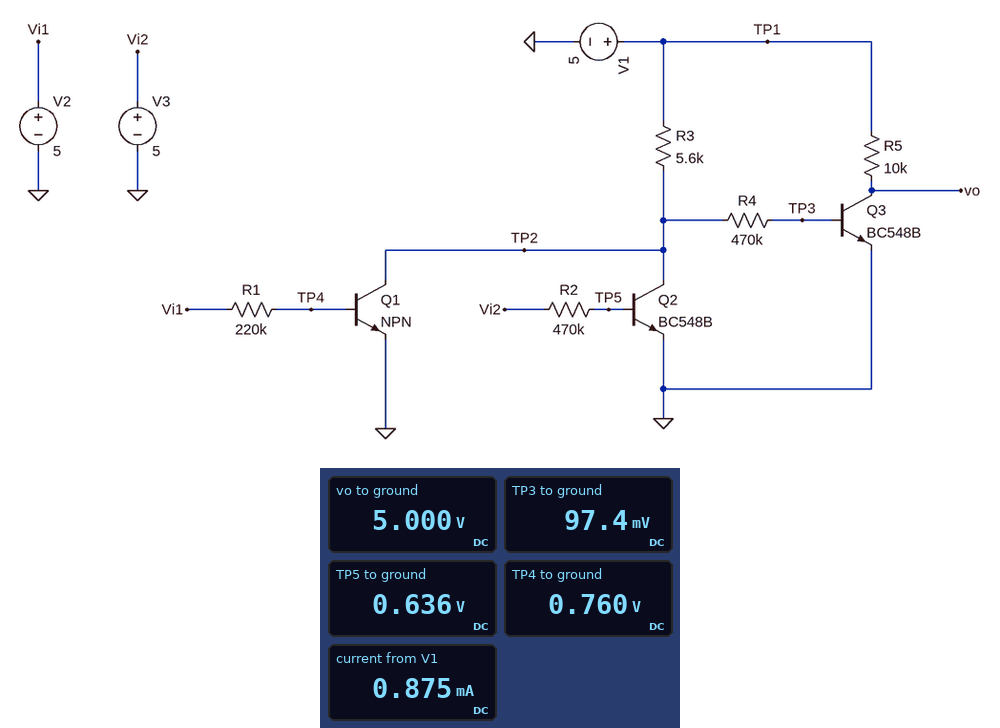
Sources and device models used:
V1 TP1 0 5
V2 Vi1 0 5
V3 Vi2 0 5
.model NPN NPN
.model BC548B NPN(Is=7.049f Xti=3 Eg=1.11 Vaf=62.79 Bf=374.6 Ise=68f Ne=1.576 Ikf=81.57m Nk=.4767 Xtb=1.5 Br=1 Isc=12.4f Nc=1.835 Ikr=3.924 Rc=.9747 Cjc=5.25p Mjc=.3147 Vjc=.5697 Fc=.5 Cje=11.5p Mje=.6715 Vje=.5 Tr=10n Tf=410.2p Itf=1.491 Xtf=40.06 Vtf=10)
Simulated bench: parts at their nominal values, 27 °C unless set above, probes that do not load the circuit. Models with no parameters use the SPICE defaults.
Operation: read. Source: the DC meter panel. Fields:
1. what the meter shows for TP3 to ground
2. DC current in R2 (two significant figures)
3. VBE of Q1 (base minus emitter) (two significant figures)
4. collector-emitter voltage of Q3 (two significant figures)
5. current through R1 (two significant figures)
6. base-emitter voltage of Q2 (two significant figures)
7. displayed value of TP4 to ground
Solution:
97.4 mV
9.3 µA
760 mV
5.0 V
19 µA
640 mV
0.760 V
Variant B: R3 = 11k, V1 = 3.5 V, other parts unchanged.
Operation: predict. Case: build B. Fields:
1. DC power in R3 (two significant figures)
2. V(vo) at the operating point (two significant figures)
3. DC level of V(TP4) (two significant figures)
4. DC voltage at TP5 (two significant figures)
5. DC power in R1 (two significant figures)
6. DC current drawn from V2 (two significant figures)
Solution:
1.1 mW
3.5 V
740 mV
610 mV
83 µW
19 µA
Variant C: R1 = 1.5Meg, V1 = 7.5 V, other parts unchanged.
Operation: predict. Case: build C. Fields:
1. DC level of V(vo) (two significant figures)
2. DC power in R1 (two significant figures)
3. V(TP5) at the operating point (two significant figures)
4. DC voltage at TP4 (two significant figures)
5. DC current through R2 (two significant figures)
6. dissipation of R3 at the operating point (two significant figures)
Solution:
7.5 V
12 µW
670 mV
730 mV
9.2 µA
9.7 mW
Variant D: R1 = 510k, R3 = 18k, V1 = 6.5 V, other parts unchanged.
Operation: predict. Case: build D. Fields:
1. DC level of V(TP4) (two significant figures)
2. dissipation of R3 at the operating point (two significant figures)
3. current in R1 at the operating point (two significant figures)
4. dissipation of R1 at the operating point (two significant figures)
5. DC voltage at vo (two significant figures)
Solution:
730 mV
2.3 mW
8.4 µA
36 µW
6.5 V
